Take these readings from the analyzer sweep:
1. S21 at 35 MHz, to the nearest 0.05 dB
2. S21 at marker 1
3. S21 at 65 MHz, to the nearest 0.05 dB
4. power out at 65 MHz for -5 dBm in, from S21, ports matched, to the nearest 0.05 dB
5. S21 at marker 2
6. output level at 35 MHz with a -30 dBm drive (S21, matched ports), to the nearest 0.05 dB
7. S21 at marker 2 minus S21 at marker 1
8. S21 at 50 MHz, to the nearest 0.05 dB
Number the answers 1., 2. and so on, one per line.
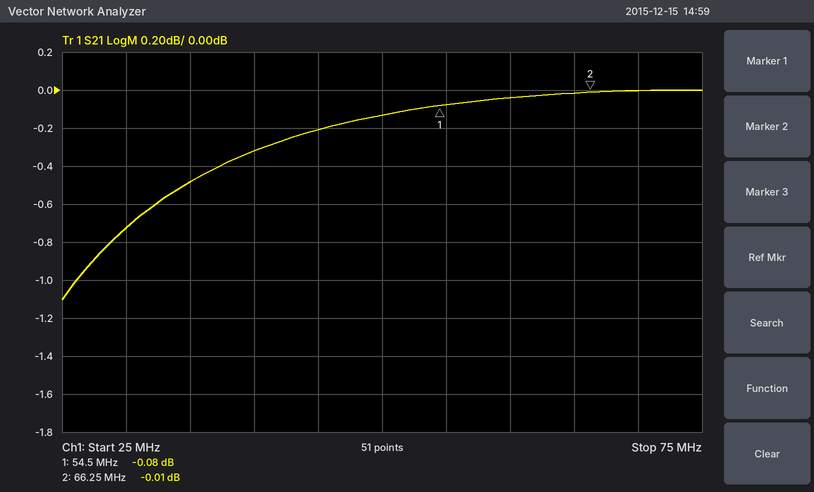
1. -0.50 dB
2. -0.08 dB
3. 0.00 dB
4. -5.00 dBm
5. -0.01 dB
6. -30.50 dBm
7. 0.07 dB
8. -0.15 dB
